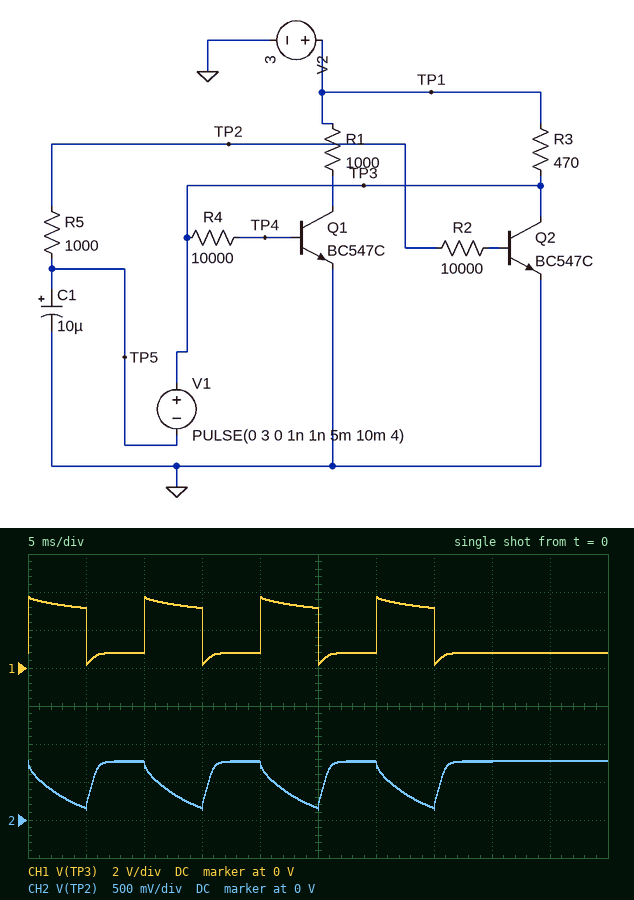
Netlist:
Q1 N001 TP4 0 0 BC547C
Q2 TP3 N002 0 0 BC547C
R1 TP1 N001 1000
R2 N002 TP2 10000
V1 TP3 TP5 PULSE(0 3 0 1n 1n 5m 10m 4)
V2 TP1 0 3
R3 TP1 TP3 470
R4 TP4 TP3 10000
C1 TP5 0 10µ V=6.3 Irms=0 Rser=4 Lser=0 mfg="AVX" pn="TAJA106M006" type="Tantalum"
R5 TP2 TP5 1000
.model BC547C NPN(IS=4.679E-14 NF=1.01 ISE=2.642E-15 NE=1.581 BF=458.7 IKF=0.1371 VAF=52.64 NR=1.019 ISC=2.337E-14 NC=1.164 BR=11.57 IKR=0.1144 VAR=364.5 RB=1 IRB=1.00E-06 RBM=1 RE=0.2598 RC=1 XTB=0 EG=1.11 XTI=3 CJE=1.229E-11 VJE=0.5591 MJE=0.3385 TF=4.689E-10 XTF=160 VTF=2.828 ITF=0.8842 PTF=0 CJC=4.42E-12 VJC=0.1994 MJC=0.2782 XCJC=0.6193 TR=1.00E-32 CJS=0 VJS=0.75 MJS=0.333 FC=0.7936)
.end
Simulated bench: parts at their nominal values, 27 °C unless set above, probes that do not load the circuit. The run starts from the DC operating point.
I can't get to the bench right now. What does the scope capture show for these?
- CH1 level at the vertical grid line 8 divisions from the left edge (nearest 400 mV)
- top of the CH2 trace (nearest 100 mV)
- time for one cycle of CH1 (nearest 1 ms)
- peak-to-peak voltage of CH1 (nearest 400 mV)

800 mV
800 mV
10 ms
3.6 V
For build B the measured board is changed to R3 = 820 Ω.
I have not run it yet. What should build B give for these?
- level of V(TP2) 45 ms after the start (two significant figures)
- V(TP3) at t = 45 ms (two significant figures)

710 mV
720 mV
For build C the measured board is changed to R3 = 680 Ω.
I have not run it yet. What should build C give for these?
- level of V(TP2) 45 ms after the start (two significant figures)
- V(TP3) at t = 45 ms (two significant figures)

730 mV
740 mV
